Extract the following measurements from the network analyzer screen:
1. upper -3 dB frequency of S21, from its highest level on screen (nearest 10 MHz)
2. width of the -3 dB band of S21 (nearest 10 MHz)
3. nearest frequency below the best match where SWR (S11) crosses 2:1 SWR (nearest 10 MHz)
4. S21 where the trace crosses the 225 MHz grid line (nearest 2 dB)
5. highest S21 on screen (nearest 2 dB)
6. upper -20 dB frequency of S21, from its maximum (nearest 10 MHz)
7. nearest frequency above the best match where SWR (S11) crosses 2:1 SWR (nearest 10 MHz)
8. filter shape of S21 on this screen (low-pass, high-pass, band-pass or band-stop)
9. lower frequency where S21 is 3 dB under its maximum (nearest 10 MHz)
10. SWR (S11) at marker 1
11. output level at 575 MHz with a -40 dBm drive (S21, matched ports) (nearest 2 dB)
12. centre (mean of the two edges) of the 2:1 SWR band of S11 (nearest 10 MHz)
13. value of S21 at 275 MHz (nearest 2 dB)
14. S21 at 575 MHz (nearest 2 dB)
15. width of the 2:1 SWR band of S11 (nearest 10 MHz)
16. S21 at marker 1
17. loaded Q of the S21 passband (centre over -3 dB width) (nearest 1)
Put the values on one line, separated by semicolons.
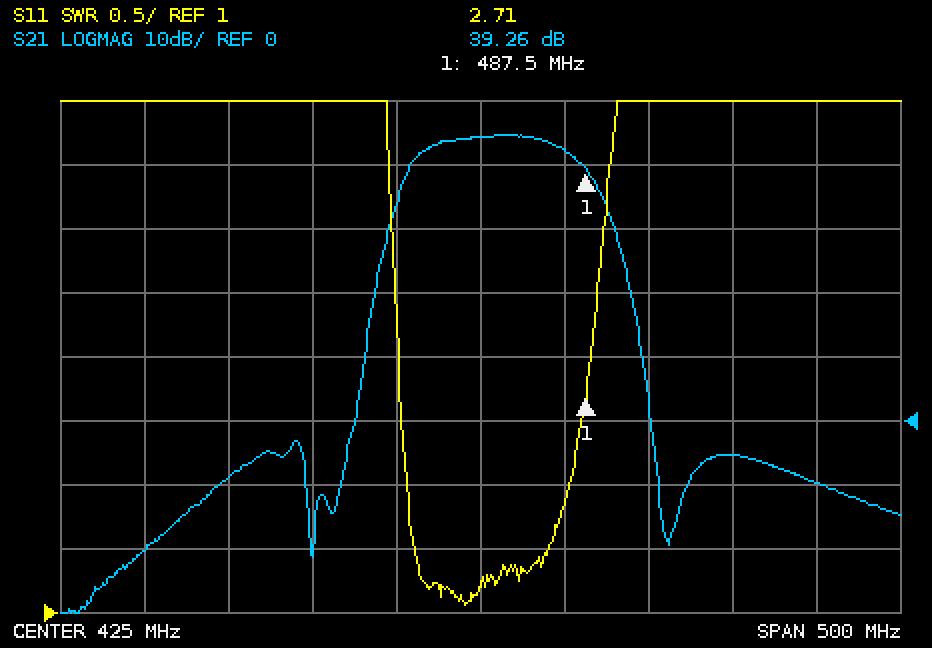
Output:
480 MHz; 90 MHz; 380 MHz; -20 dB; 44 dB; 510 MHz; 480 MHz; band-pass; 390 MHz; 2.71; -46 dBm; 430 MHz; -8 dB; -6 dB; 100 MHz; 39.26 dB; 5
